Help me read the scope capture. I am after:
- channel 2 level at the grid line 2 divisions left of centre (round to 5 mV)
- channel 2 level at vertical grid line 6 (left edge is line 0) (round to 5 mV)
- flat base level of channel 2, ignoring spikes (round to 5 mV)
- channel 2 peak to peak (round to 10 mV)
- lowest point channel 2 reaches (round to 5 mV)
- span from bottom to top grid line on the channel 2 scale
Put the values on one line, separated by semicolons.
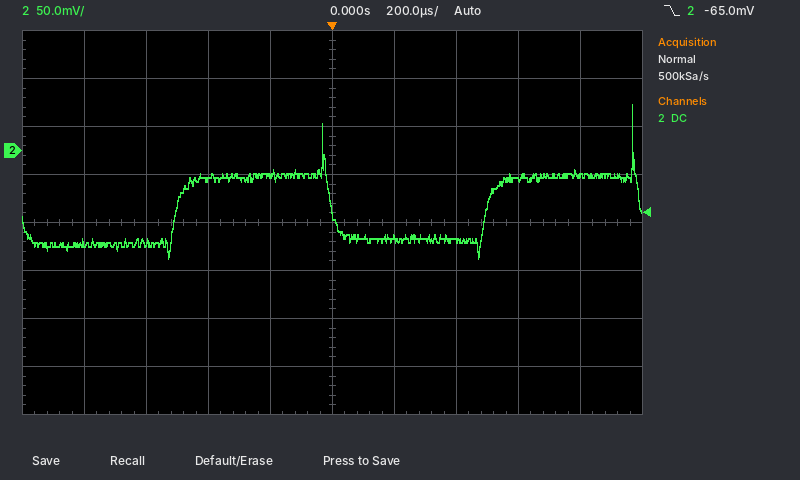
-30 mV; -90 mV; -95 mV; 160 mV; -110 mV; 400 mV
